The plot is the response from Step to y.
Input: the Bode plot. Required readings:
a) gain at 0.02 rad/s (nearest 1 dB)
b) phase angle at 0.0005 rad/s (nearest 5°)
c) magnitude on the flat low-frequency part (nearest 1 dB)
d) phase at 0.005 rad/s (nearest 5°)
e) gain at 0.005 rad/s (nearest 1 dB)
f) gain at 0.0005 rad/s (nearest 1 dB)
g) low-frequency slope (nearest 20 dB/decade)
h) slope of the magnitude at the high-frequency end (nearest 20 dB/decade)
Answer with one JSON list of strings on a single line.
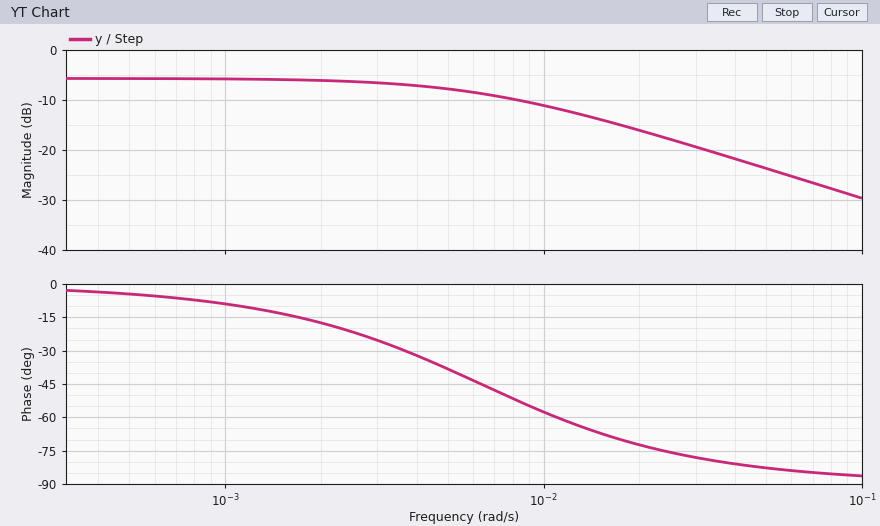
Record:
["-16 dB", "-5°", "-6 dB", "-40°", "-8 dB", "-6 dB", "0 dB/decade", "-20 dB/decade"]
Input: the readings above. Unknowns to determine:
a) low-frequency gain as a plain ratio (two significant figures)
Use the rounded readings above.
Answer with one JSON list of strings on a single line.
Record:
["0.50"]
